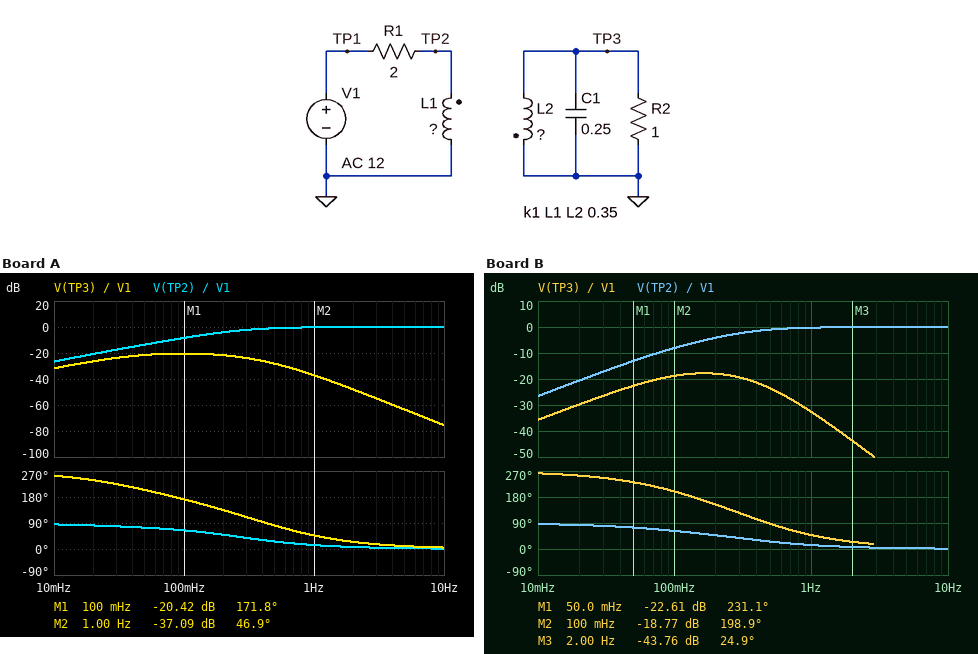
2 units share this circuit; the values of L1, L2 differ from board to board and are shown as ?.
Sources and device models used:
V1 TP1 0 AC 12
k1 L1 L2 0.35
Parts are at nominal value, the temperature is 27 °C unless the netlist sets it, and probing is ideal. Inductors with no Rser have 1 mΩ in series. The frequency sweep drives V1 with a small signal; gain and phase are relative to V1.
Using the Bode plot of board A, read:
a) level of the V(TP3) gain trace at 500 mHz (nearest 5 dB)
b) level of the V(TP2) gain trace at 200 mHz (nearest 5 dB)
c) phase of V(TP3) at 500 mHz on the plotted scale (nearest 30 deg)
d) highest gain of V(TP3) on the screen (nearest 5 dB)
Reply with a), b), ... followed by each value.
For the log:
a) -30 dB
b) -5 dB
c) 90 deg
d) -20 dB
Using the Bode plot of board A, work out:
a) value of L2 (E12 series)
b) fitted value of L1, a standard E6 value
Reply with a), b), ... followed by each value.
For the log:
a) 3.9 H
b) 1.5 H
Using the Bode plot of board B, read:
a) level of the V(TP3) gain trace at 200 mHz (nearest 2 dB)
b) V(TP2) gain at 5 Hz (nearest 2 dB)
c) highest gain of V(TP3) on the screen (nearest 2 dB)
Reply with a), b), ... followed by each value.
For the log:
a) -18 dB
b) 0 dB
c) -18 dB
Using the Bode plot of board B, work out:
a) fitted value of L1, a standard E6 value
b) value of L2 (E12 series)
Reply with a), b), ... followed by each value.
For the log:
a) 1.5 H
b) 1.5 H
